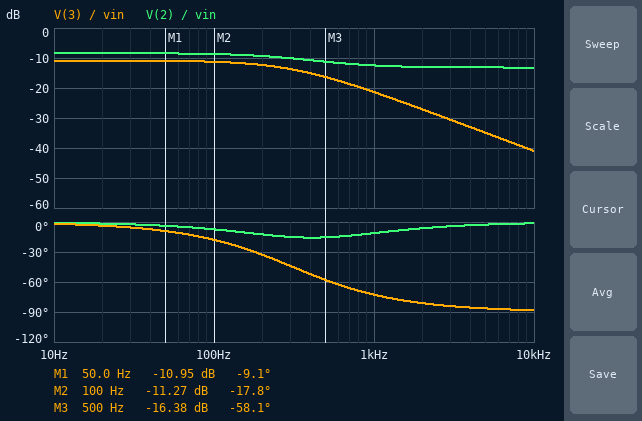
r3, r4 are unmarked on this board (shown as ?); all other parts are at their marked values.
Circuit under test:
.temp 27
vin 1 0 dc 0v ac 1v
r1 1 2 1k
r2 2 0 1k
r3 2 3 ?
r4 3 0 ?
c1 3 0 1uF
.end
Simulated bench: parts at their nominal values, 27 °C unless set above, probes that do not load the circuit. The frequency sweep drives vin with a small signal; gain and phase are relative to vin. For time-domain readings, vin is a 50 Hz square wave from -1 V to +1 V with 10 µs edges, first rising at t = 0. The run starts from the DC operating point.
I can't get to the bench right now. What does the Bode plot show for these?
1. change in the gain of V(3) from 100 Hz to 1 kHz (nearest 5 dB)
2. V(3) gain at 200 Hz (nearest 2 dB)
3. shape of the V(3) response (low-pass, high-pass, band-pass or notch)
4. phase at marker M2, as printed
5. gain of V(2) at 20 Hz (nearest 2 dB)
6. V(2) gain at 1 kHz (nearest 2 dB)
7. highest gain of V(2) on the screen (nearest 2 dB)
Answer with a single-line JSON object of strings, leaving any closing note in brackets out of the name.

{"change in the gain of V(3) from 100 Hz to 1 kHz": "-10 dB", "V(3) gain at 200 Hz": "-12 dB", "shape of the V(3) response": "low-pass", "phase at marker M2, as printed": "-17.8 deg", "gain of V(2) at 20 Hz": "-8 dB", "V(2) gain at 1 kHz": "-12 dB", "highest gain of V(2) on the screen": "-8 dB"}
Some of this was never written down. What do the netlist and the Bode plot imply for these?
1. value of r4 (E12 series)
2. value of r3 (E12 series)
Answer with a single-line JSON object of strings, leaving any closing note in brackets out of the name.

{"value of r4": "1.2 kΩ", "value of r3": "390 Ω"}
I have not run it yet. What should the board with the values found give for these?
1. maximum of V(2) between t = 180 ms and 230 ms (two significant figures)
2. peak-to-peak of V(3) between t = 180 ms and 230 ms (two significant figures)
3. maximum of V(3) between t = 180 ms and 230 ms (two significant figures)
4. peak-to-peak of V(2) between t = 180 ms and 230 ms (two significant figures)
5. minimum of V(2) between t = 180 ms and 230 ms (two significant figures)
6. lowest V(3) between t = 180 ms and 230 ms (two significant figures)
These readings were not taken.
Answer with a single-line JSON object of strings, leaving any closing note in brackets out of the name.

{"maximum of V(2) between t = 180 ms and 230 ms": "380 mV", "peak-to-peak of V(3) between t = 180 ms and 230 ms": "570 mV", "maximum of V(3) between t = 180 ms and 230 ms": "290 mV", "peak-to-peak of V(2) between t = 180 ms and 230 ms": "760 mV", "minimum of V(2) between t = 180 ms and 230 ms": "-380 mV", "lowest V(3) between t = 180 ms and 230 ms": "-290 mV"}
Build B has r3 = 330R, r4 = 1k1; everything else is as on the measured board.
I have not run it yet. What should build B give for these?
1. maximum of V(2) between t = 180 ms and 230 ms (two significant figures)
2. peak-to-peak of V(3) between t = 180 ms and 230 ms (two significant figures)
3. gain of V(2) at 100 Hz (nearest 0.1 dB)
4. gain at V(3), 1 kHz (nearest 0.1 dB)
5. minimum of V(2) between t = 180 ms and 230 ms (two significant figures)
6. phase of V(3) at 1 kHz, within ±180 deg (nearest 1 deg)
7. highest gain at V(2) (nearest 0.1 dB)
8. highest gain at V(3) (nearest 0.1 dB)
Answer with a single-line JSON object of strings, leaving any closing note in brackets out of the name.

{"maximum of V(2) between t = 180 ms and 230 ms": "370 mV", "peak-to-peak of V(3) between t = 180 ms and 230 ms": "570 mV", "gain of V(2) at 100 Hz": "-8.9 dB", "gain at V(3), 1 kHz": "-20.8 dB", "minimum of V(2) between t = 180 ms and 230 ms": "-370 mV", "phase of V(3) at 1 kHz, within ±180 deg": "-71 deg", "highest gain at V(2)": "-8.6 dB", "highest gain at V(3)": "-10.9 dB"}
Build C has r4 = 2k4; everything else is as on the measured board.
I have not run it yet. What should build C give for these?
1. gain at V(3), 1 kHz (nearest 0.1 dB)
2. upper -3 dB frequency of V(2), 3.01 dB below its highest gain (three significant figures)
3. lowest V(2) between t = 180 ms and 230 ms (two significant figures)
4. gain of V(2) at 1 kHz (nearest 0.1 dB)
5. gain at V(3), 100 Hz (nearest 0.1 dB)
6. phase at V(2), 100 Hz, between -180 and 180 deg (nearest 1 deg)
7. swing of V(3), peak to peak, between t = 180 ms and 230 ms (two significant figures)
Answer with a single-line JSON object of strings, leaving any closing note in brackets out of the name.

{"gain at V(3), 1 kHz": "-21.2 dB", "upper -3 dB frequency of V(2), 3.01 dB below its highest gain": "359 Hz", "lowest V(2) between t = 180 ms and 230 ms": "-420 mV", "gain of V(2) at 1 kHz": "-12.6 dB", "gain at V(3), 100 Hz": "-9.4 dB", "phase at V(2), 100 Hz, between -180 and 180 deg": "-10 deg", "swing of V(3), peak to peak, between t = 180 ms and 230 ms": "730 mV"}
